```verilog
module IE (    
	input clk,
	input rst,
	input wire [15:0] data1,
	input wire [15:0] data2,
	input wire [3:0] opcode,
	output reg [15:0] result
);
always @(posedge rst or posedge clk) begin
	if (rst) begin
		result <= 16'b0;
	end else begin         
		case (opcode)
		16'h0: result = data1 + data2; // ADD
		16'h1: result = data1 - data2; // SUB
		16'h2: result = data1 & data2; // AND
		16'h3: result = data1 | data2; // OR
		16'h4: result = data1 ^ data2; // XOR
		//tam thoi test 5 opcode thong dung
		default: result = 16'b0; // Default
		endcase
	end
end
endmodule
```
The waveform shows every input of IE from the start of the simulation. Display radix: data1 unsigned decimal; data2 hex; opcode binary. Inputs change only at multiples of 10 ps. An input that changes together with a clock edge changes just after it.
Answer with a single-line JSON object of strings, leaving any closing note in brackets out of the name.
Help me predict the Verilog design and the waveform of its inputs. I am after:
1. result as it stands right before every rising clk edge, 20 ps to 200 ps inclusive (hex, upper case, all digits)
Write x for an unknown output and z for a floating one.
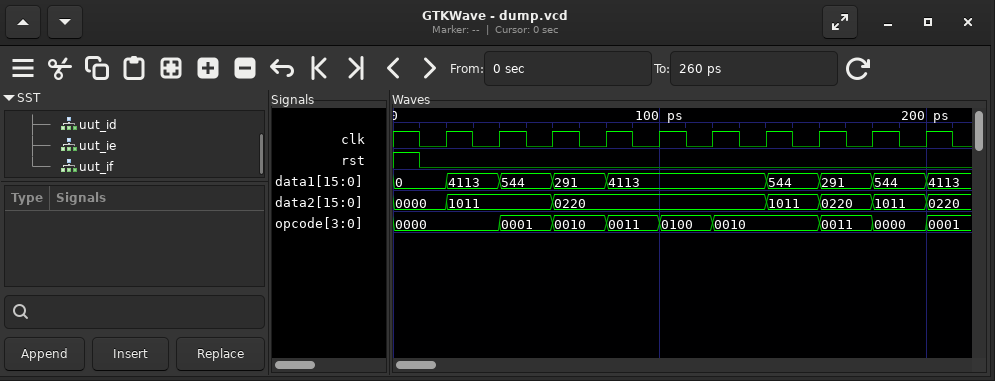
{"result as it stands right before every rising clk edge, 20 ps to 200 ps inclusive": "0000, 0000, 2022, F20F, 0020, 1231, 1231, 0000, 0000, 0323"}
